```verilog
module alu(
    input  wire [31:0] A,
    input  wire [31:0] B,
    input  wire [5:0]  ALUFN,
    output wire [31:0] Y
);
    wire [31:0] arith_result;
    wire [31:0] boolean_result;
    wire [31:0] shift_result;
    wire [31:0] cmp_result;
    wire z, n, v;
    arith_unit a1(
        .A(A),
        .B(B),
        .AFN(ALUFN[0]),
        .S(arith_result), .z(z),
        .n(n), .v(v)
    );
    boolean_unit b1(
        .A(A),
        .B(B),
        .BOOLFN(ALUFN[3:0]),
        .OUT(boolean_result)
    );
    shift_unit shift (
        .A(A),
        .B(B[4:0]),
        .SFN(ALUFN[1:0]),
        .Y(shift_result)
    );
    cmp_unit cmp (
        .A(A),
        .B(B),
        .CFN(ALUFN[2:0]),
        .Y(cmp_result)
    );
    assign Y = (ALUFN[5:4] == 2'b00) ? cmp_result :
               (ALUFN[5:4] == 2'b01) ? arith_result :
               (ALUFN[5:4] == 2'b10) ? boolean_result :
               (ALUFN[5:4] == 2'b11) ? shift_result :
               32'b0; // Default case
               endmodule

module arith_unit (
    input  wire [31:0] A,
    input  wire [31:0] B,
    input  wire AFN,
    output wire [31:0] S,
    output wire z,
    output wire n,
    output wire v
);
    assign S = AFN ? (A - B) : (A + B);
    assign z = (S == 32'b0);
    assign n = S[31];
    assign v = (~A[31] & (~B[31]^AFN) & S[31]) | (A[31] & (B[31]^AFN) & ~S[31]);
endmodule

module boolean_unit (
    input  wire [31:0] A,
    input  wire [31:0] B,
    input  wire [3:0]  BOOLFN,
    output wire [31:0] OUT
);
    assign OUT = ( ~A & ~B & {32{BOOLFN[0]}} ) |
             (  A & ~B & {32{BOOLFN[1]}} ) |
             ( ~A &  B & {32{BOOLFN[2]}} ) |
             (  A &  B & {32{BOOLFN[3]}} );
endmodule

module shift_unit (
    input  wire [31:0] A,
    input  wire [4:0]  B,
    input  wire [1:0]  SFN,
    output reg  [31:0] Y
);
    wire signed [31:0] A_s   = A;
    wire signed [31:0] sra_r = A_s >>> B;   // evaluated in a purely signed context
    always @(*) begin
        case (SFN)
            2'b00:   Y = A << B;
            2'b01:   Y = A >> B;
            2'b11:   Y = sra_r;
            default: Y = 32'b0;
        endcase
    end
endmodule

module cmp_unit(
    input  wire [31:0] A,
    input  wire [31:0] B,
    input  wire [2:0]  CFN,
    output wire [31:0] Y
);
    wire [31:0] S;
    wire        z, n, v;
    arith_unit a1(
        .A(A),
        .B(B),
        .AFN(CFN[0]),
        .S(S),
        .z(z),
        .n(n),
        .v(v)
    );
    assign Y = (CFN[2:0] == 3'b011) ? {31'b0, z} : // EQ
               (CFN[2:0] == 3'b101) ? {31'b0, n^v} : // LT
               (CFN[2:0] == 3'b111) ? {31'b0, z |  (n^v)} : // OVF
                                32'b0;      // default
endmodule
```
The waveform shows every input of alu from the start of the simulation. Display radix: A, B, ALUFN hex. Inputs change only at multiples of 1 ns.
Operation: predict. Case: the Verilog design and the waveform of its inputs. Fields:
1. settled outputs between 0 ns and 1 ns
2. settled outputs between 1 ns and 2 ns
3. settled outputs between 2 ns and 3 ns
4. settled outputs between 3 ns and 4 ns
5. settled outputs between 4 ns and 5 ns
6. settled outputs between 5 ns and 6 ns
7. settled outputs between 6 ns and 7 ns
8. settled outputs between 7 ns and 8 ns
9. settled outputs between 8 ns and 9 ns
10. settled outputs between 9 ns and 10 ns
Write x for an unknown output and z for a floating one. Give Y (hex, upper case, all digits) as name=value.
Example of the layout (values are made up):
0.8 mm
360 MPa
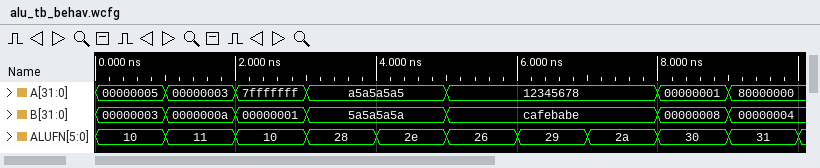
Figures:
Y=00000008
Y=FFFFFFF9
Y=80000000
Y=00000000
Y=FFFFFFFF
Y=D8CAECC6
Y=27351339
Y=12345678
Y=00000100
Y=08000000
